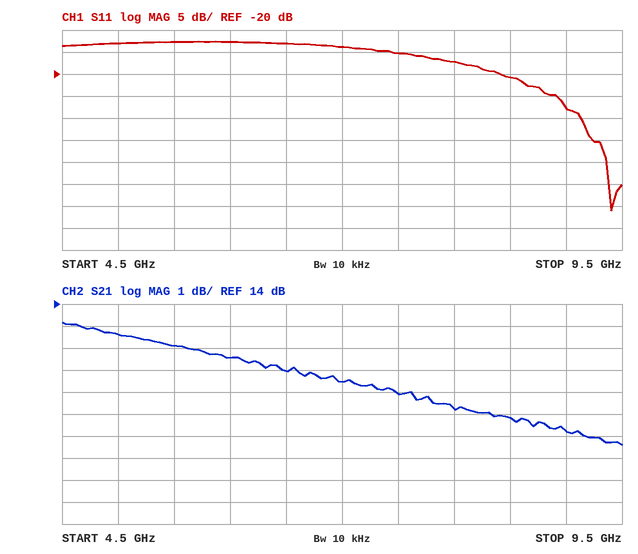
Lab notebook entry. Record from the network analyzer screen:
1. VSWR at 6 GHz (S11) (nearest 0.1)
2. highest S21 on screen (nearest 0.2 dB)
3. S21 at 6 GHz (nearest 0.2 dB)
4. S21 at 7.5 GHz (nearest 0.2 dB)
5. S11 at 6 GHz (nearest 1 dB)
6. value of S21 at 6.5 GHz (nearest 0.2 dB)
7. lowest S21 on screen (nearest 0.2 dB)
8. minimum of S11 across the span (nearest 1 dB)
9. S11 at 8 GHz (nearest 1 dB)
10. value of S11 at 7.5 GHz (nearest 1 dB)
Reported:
1.6
13.2 dB
11.6 dB
10.0 dB
-13 dB
11.0 dB
7.6 dB
-51 dB
-17 dB
-15 dB
